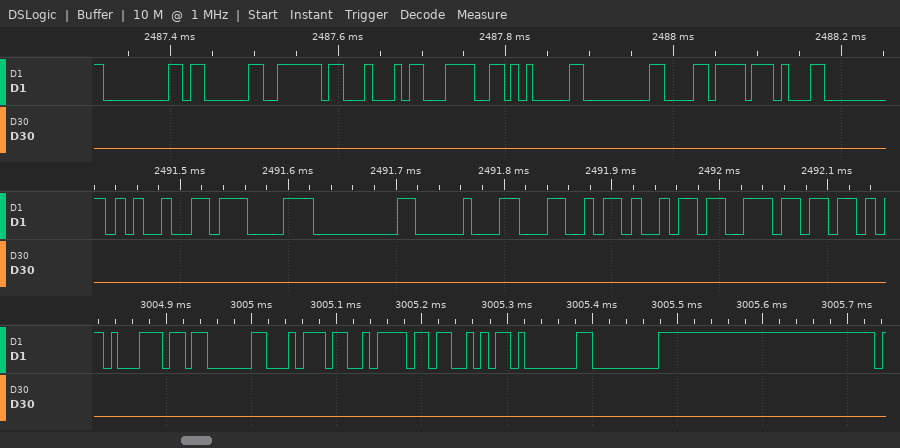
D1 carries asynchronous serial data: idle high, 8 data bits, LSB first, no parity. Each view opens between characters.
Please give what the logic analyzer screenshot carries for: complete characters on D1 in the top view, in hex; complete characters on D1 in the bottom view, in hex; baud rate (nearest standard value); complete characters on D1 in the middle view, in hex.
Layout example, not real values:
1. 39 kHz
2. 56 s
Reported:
1. 00, 03, 7E, 44, 3C, 05, 00, D8, 17
2. 71, 03, 74, 7A, 53, 01, 00
3. 115200 baud
4. 25, 87, 00, 10, 4C, 69, 6E
